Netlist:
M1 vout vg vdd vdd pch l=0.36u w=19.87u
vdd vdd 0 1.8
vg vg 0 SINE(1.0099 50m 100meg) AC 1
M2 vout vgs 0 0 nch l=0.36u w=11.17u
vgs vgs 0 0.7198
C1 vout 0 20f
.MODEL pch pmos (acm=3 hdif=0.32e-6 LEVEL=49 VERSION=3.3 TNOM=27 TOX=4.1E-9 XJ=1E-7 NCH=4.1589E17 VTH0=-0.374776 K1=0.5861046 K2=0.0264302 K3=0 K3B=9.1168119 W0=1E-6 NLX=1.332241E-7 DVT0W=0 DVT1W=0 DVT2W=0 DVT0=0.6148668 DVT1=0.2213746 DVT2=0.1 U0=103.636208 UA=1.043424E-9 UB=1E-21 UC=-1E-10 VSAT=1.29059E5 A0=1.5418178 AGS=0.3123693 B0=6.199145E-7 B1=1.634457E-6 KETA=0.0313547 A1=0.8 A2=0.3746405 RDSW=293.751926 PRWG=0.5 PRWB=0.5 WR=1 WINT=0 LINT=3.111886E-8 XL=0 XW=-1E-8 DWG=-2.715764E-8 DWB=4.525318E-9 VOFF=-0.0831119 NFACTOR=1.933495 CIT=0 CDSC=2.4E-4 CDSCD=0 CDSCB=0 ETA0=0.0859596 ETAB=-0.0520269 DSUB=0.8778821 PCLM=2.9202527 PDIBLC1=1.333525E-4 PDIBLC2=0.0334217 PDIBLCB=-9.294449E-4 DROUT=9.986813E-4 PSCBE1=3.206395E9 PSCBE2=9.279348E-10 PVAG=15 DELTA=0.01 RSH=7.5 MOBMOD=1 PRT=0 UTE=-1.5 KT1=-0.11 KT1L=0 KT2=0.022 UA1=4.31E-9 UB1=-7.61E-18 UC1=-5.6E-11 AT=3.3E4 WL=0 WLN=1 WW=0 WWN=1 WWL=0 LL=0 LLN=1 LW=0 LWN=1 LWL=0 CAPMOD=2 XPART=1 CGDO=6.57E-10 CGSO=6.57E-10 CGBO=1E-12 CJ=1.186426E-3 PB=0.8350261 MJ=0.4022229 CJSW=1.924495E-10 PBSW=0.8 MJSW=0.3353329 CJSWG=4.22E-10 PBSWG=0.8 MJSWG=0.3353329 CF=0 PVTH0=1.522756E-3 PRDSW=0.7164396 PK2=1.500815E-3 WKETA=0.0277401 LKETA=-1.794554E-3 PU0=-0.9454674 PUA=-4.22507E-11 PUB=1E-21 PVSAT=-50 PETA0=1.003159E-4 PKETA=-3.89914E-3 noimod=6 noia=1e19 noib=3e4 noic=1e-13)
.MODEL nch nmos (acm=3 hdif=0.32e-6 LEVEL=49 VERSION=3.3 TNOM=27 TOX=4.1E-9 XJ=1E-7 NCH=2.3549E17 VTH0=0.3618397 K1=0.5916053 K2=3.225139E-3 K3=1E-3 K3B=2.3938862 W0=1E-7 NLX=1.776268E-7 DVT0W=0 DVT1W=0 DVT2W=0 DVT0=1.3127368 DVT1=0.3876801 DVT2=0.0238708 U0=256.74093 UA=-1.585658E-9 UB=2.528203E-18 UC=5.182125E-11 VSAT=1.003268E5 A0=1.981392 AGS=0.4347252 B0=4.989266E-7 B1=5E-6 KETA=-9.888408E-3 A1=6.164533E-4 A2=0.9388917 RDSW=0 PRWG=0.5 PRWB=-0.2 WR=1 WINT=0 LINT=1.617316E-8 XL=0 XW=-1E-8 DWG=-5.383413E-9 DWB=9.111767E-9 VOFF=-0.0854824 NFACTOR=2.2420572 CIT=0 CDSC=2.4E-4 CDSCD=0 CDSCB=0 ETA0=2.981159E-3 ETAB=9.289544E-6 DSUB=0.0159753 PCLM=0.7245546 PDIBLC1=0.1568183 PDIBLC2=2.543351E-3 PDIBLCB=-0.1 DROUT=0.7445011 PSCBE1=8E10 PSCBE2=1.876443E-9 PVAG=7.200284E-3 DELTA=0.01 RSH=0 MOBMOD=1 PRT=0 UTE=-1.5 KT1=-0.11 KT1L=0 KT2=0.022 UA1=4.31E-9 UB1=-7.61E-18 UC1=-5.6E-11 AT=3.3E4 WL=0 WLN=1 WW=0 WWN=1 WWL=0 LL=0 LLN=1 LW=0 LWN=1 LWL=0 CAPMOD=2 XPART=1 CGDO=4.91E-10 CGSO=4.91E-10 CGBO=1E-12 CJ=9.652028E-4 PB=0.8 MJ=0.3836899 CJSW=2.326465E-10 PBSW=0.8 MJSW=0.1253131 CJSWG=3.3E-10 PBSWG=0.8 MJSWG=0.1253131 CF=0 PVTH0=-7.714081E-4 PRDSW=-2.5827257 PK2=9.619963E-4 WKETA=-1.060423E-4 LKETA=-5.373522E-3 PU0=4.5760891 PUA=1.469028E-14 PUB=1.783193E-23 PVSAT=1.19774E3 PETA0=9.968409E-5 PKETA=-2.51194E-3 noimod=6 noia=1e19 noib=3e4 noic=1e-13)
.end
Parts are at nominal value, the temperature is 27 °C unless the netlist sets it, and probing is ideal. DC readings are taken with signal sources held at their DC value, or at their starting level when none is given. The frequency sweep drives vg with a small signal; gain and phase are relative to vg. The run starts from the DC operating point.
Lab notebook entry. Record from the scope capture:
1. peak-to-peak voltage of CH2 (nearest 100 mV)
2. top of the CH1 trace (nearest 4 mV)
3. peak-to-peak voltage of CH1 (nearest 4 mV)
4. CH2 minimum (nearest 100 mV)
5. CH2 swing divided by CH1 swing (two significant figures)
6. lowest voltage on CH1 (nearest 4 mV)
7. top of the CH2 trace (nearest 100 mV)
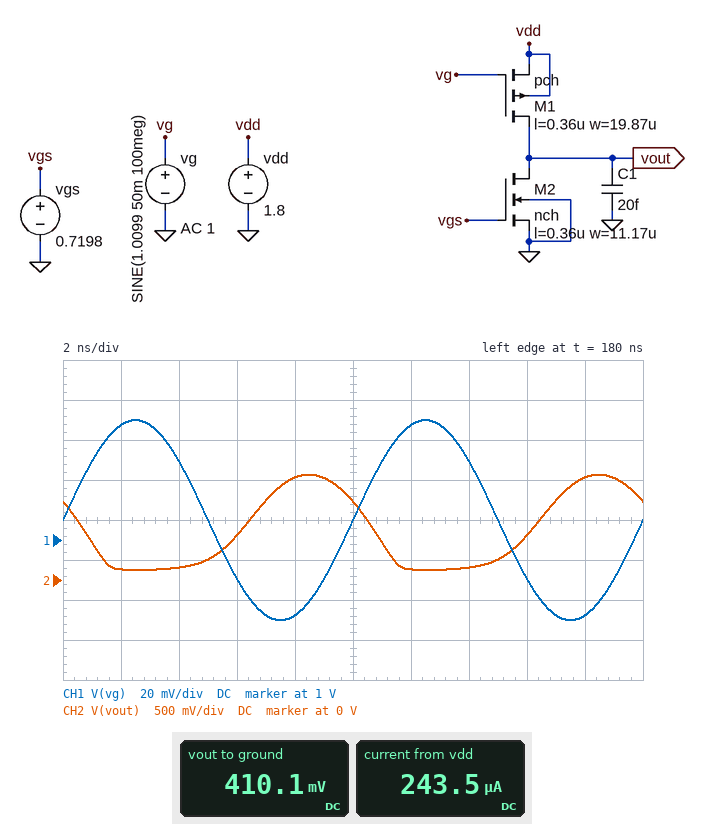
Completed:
1.2 V
1.060 V
100 mV
100 mV
12
960 mV
1.3 V
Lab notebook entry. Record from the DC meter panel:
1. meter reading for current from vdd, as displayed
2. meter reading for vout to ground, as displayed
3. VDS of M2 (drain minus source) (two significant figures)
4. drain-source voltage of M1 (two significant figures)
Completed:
243.5 µA
410.1 mV
410 mV
-1.4 V
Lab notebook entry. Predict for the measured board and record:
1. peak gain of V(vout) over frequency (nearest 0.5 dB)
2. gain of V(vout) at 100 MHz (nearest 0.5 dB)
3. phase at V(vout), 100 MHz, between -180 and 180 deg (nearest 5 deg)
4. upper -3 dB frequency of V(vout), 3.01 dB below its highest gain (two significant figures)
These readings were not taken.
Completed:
26.0 dB
24.0 dB
145 deg
150 MHz
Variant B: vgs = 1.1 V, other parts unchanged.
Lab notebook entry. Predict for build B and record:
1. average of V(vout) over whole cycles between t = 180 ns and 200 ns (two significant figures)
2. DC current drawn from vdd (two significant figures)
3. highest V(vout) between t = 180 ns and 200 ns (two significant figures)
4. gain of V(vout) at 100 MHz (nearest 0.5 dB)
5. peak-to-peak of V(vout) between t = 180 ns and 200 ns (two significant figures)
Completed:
45 mV
250 µA
58 mV
-12.0 dB
25 mV
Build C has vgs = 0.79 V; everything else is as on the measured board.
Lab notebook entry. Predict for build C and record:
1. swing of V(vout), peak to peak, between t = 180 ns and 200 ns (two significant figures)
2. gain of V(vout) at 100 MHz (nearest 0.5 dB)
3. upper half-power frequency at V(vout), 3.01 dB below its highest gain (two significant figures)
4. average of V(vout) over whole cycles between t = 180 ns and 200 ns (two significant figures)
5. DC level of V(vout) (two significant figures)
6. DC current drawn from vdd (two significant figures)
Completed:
89 mV
-1.5 dB
2.8 GHz
120 mV
110 mV
250 µA
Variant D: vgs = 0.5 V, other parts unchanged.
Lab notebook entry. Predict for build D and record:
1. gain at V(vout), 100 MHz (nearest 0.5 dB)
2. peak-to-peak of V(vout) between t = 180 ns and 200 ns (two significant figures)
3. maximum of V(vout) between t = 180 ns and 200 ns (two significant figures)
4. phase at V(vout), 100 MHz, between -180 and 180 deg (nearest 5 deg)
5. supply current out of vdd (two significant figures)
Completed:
-28.0 dB
4.2 mV
1.8 V
150 deg
17 µA
